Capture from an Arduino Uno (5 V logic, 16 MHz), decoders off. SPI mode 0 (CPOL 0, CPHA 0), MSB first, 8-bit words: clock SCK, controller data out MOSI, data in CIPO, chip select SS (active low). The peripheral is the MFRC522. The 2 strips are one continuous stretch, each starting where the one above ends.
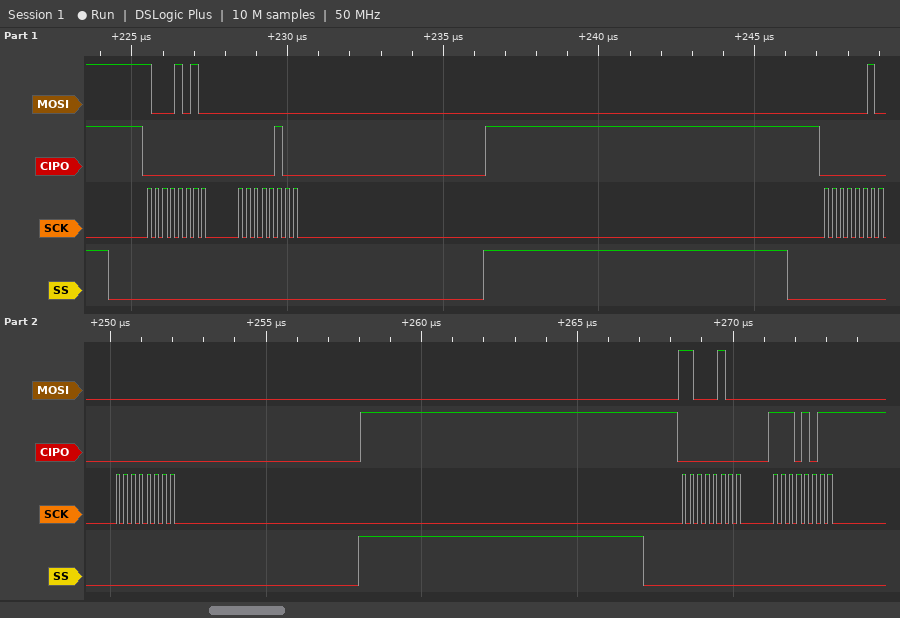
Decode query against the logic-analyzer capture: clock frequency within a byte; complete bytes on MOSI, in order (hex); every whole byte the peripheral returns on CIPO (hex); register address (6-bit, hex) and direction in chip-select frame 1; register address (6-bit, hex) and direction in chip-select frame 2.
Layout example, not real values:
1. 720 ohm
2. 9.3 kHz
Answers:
1. 4 MHz
2. 8A 00 02 00 C4 00
3. 00 04 00 00 00 EB
4. 0x05 read
5. 0x01 write
